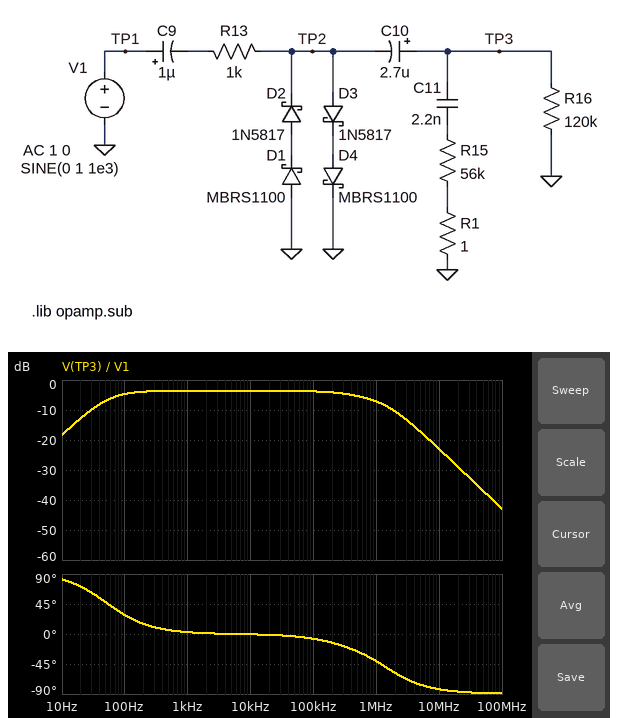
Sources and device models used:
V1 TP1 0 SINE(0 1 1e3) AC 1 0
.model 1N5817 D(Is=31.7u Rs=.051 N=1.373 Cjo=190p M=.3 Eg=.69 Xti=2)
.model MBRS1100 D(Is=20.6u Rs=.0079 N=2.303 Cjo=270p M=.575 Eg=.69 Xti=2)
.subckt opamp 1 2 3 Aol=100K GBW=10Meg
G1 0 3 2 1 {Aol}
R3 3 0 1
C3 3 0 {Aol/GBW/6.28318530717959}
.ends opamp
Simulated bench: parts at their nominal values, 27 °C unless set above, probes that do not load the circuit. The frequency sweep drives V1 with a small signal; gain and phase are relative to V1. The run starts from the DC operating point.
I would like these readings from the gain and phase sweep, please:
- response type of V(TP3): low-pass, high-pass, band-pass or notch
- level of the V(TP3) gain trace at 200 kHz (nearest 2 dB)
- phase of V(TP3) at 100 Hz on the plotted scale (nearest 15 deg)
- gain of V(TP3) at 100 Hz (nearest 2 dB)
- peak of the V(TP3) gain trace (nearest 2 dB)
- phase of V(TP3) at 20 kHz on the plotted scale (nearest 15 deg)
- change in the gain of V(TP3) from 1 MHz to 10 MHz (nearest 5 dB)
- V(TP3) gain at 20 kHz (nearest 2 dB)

band-pass
-4 dB
30 deg
-4 dB
-4 dB
0 deg
-15 dB
-4 dB
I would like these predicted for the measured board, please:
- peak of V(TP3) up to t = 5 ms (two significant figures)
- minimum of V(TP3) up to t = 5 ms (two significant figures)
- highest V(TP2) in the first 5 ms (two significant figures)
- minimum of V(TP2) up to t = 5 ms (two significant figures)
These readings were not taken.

320 mV
-320 mV
320 mV
-320 mV
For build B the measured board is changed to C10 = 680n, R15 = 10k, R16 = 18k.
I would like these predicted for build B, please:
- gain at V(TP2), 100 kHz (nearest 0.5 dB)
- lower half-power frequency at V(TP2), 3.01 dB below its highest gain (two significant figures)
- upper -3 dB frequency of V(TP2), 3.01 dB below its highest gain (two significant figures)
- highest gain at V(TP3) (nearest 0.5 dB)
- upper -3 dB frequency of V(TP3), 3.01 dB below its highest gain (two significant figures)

-4.5 dB
57 Hz
800 kHz
-4.0 dB
810 kHz
